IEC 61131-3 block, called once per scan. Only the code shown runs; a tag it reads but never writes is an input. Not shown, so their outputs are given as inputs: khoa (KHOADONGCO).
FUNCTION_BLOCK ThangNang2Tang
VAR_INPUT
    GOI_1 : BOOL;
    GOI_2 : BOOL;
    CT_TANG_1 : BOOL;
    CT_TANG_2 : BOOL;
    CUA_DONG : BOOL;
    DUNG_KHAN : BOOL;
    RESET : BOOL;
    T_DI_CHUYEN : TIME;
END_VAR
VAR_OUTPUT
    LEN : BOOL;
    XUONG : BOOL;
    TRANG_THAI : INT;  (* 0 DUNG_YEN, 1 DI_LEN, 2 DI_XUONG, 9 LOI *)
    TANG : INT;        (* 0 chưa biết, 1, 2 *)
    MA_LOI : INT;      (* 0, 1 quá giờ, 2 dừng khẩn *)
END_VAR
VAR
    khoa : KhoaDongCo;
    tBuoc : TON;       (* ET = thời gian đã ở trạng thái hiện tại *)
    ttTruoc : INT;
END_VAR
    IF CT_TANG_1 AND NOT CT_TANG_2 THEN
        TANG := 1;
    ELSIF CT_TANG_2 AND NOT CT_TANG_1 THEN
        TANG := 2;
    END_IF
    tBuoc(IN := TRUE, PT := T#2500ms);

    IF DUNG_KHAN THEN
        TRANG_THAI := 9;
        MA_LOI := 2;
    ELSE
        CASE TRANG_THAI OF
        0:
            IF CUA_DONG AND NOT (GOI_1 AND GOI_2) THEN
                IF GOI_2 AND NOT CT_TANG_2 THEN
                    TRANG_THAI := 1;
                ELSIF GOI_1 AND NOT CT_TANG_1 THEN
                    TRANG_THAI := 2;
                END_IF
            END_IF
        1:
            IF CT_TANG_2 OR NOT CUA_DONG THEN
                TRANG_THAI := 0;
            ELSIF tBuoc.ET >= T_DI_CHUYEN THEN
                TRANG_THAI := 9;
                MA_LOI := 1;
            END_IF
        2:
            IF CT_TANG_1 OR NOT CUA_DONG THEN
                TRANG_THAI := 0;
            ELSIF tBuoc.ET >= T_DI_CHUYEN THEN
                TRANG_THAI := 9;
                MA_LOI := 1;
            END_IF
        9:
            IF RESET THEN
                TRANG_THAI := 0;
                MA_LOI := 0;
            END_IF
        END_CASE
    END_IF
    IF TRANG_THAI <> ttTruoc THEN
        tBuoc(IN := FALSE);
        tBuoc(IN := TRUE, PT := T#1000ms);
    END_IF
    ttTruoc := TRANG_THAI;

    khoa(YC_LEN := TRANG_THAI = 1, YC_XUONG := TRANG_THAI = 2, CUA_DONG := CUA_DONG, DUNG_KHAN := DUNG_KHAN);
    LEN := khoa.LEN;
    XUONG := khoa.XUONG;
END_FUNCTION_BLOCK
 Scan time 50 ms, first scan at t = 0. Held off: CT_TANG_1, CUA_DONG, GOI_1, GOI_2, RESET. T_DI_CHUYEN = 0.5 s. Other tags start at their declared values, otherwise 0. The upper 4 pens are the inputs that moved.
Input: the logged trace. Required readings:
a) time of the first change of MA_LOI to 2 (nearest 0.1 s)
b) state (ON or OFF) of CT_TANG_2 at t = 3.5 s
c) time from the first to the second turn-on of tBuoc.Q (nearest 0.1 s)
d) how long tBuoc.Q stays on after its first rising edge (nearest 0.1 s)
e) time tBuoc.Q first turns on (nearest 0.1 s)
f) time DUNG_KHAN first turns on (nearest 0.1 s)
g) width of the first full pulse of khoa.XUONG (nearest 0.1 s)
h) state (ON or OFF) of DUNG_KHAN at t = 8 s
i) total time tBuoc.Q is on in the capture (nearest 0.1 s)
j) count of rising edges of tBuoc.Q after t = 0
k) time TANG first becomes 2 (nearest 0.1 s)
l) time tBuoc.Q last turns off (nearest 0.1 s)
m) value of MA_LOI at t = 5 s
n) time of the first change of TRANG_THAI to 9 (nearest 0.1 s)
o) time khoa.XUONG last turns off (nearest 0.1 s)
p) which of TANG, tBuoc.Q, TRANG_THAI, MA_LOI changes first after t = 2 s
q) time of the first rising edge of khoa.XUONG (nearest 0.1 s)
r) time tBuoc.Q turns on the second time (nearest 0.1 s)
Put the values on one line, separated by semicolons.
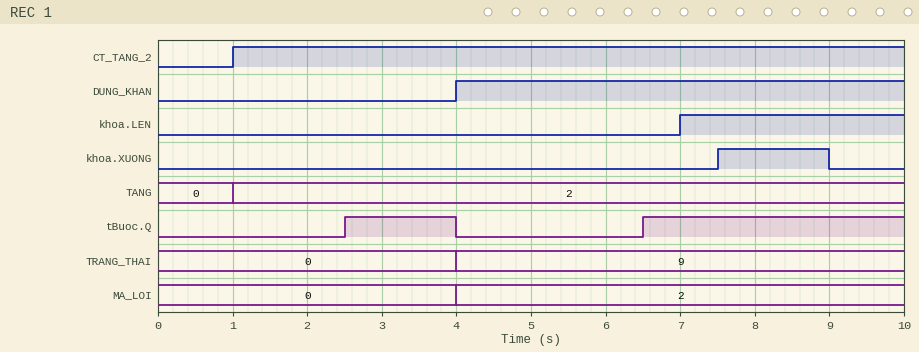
4.0 s; ON; 4.0 s; 1.5 s; 2.5 s; 4.0 s; 1.5 s; ON; 5.0 s; 2; 1.0 s; 4.0 s; 2; 4.0 s; 9.0 s; tBuoc.Q; 7.5 s; 6.5 s
